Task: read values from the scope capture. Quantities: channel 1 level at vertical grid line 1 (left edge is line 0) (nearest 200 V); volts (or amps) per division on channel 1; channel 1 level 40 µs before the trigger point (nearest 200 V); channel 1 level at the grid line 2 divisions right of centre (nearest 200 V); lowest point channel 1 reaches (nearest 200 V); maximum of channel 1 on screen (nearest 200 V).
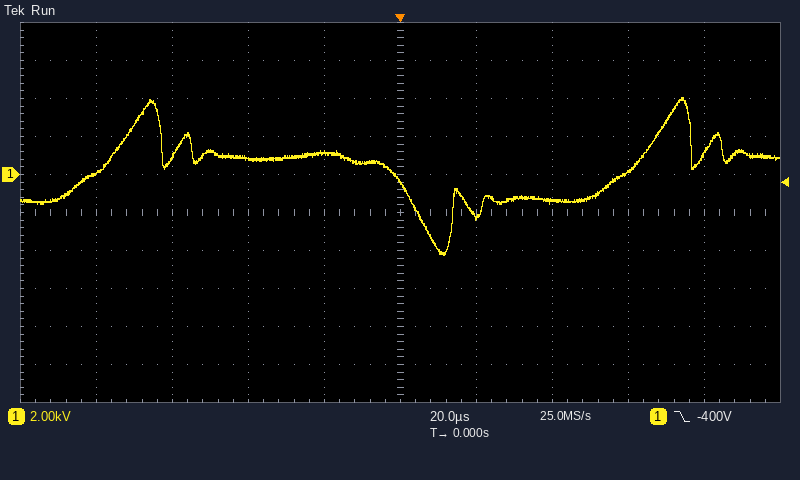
0.0 kV
2 kV
800 V
-1.4 kV
-4.2 kV
4.0 kV
